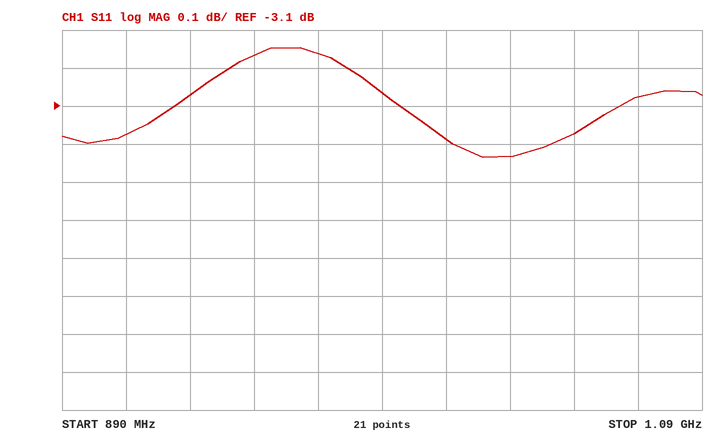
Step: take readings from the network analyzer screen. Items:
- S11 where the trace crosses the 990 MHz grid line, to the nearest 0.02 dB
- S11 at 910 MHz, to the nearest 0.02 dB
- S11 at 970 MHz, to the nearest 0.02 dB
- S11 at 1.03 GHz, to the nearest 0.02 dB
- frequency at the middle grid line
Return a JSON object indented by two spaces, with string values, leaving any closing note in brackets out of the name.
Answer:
{
  "S11 where the trace crosses the 990 MHz grid line, to the nearest 0.02 dB": "-3.06 dB",
  "S11 at 910 MHz, to the nearest 0.02 dB": "-3.18 dB",
  "S11 at 970 MHz, to the nearest 0.02 dB": "-2.96 dB",
  "S11 at 1.03 GHz, to the nearest 0.02 dB": "-3.24 dB",
  "frequency at the middle grid line": "990 MHz"
}
